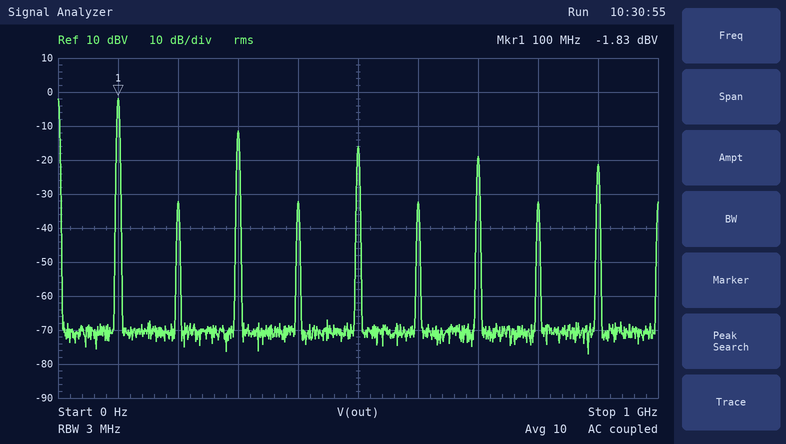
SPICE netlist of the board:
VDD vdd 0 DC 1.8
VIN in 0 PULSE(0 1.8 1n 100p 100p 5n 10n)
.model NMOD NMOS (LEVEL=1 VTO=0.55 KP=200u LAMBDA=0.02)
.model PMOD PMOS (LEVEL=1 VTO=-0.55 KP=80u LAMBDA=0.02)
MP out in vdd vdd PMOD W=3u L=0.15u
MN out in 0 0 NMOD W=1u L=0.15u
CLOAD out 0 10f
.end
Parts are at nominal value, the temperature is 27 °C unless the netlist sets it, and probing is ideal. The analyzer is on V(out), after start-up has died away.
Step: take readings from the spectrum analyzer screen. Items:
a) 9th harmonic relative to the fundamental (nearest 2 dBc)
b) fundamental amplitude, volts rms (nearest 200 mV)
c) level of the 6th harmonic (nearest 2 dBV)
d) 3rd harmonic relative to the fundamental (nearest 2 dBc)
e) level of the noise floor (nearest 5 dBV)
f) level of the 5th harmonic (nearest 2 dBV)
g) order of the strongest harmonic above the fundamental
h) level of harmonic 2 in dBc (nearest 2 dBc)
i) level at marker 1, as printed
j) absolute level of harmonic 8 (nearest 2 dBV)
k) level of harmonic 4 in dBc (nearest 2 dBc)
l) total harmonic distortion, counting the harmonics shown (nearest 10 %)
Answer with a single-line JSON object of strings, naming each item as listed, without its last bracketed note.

{"9th harmonic relative to the fundamental": "-20 dBc", "fundamental amplitude, volts rms": "800 mV", "level of the 6th harmonic": "-32 dBV", "3rd harmonic relative to the fundamental": "-10 dBc", "level of the noise floor": "-70 dBV", "level of the 5th harmonic": "-16 dBV", "order of the strongest harmonic above the fundamental": "3", "level of harmonic 2 in dBc": "-30 dBc", "level at marker 1, as printed": "-1.83 dBV", "absolute level of harmonic 8": "-32 dBV", "level of harmonic 4 in dBc": "-30 dBc", "total harmonic distortion, counting the harmonics shown": "40 %"}
